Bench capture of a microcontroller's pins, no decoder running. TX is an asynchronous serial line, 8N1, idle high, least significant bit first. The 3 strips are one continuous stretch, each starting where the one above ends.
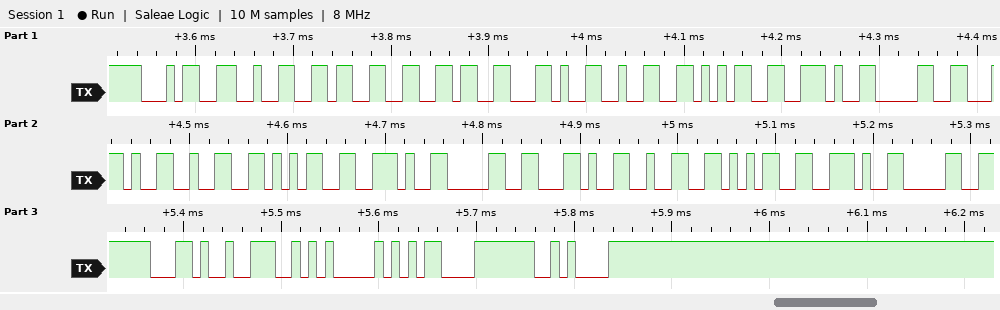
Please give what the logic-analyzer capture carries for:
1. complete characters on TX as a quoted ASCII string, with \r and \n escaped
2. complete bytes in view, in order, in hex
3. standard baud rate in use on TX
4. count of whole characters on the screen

"4236,25.0,25.0,25.0,NA\r\n"
34 32 33 36 2C 32 35 2E 30 2C 32 35 2E 30 2C 32 35 2E 30 2C 4E 41 0D 0A
115200 baud
24
